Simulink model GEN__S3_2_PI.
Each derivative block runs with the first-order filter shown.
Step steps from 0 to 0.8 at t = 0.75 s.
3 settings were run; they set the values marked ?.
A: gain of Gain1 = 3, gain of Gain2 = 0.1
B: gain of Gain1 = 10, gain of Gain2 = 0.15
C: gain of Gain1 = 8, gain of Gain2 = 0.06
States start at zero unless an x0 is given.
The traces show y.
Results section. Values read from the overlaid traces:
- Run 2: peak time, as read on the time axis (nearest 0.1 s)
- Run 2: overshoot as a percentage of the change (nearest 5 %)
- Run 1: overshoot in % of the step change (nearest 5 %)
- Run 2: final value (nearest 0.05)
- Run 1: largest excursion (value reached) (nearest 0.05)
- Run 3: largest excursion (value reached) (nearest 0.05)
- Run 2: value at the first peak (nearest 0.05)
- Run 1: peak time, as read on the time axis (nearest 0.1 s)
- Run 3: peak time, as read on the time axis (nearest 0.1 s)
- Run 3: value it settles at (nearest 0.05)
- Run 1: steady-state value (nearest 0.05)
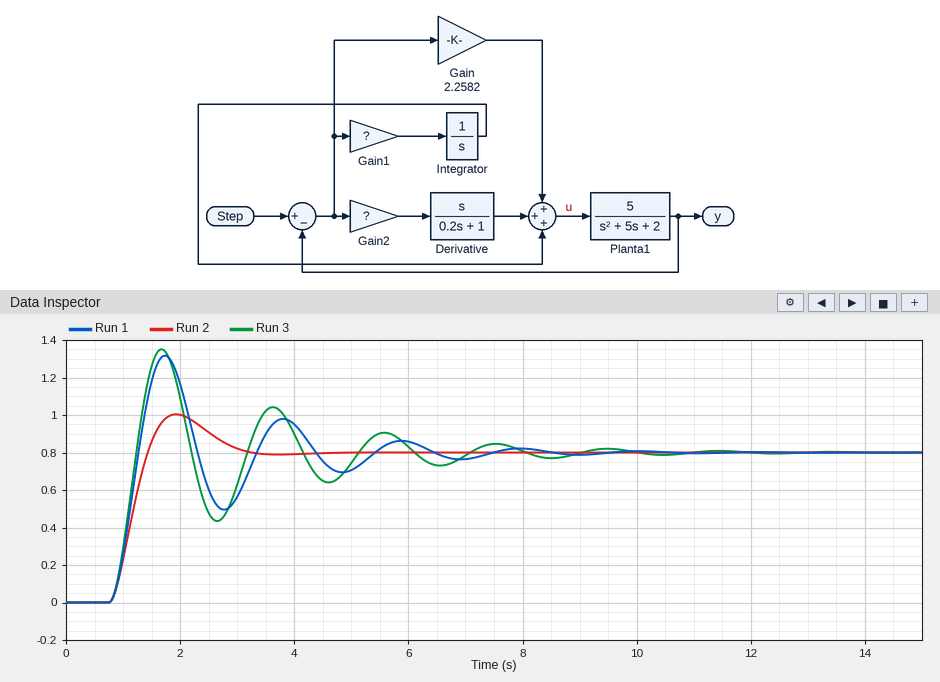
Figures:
1.9 s
25 %
65 %
0.80
1.30
1.35
1.00
1.7 s
1.7 s
0.80
0.80
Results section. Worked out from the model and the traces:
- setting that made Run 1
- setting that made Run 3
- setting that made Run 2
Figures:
C
B
A
